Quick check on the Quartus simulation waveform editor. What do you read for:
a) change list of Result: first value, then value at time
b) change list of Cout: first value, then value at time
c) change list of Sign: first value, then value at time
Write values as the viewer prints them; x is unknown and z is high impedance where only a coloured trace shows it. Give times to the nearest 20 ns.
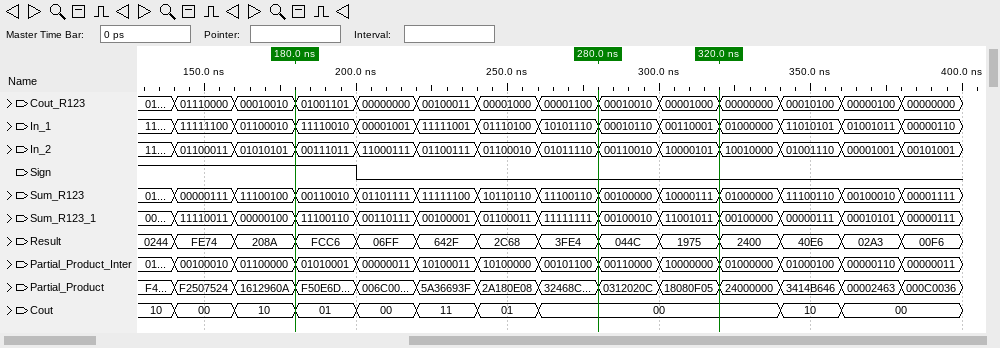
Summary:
0244, FE74 at 140 ns, 208A at 160 ns, FCC6 at 180 ns, 06FF at 200 ns, 642F at 220 ns, 2C68 at 240 ns, 3FE4 at 260 ns, 044C at 280 ns, 1975 at 300 ns, 2400 at 320 ns, 40E6 at 340 ns, 02A3 at 360 ns, 00F6 at 380 ns
10, 00 at 140 ns, 10 at 160 ns, 01 at 180 ns, 00 at 200 ns, 11 at 220 ns, 01 at 240 ns, 00 at 260 ns, 10 at 340 ns, 00 at 360 ns
1, 0 at 200 ns
